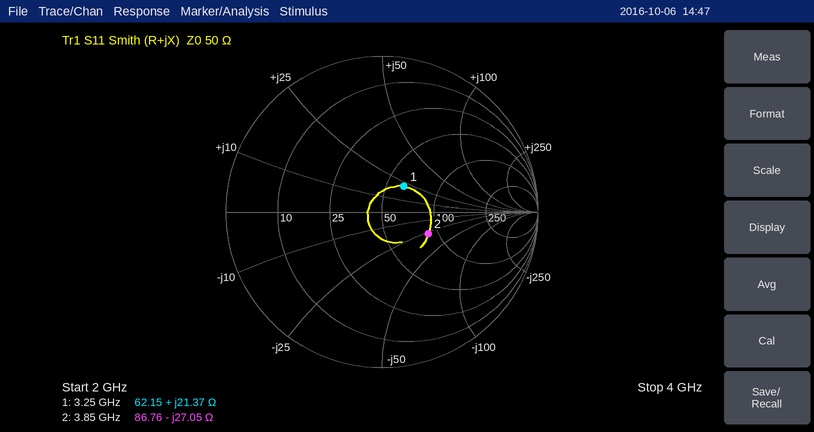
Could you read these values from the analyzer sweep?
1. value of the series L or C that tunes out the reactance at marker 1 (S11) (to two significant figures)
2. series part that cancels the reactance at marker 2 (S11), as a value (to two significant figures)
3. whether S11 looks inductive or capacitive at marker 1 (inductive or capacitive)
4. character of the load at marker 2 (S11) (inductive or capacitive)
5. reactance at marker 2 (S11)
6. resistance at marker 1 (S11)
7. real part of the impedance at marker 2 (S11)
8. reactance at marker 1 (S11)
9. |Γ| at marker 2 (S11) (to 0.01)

2.3 pF
1.1 nH
inductive
capacitive
-27.05 Ω
62.15 Ω
86.76 Ω
+21.37 Ω
0.33
